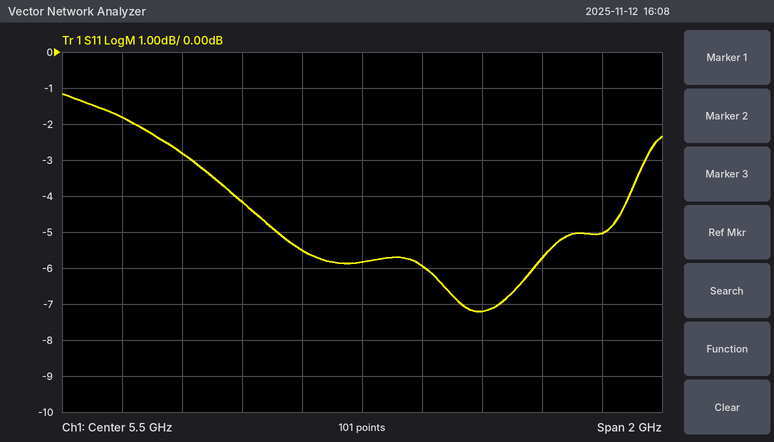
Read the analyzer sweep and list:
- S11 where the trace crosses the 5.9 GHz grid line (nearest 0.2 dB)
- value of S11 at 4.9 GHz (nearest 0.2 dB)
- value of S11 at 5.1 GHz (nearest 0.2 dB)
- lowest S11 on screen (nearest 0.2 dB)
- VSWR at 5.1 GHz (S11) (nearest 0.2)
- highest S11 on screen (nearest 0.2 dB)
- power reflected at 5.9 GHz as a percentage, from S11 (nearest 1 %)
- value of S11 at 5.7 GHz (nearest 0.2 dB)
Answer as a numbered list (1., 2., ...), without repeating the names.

1. -7.2 dB
2. -2.8 dB
3. -4.2 dB
4. -7.2 dB
5. 4.2
6. -1.2 dB
7. 19 %
8. -6.0 dB
